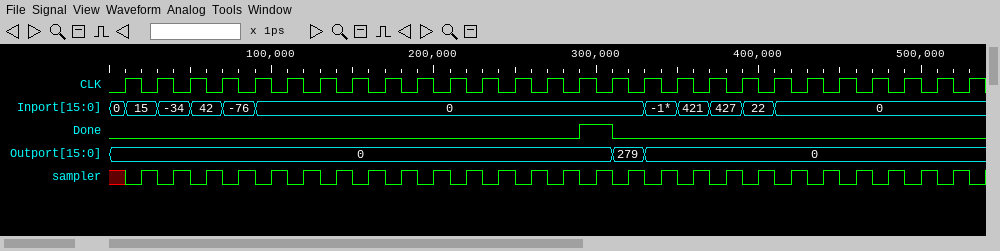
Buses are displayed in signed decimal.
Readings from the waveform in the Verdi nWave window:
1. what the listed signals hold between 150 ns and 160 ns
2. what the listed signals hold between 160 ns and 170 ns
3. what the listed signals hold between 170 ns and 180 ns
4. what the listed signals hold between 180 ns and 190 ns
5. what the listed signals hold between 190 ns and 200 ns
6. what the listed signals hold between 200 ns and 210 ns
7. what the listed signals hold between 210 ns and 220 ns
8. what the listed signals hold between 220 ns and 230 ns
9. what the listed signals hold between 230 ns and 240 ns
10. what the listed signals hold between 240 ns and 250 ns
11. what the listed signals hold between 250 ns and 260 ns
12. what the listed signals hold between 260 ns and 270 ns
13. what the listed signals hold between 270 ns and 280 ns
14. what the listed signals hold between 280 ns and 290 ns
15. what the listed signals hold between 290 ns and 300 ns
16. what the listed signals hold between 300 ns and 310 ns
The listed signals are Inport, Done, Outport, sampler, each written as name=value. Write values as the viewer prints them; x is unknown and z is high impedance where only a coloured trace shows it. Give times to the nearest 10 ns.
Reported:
Inport=0, Done=0, Outport=0, sampler=0
Inport=0, Done=0, Outport=0, sampler=1
Inport=0, Done=0, Outport=0, sampler=0
Inport=0, Done=0, Outport=0, sampler=1
Inport=0, Done=0, Outport=0, sampler=0
Inport=0, Done=0, Outport=0, sampler=1
Inport=0, Done=0, Outport=0, sampler=0
Inport=0, Done=0, Outport=0, sampler=1
Inport=0, Done=0, Outport=0, sampler=0
Inport=0, Done=0, Outport=0, sampler=1
Inport=0, Done=0, Outport=0, sampler=0
Inport=0, Done=0, Outport=0, sampler=1
Inport=0, Done=0, Outport=0, sampler=0
Inport=0, Done=0, Outport=0, sampler=1
Inport=0, Done=1, Outport=0, sampler=0
Inport=0, Done=1, Outport=0, sampler=1
